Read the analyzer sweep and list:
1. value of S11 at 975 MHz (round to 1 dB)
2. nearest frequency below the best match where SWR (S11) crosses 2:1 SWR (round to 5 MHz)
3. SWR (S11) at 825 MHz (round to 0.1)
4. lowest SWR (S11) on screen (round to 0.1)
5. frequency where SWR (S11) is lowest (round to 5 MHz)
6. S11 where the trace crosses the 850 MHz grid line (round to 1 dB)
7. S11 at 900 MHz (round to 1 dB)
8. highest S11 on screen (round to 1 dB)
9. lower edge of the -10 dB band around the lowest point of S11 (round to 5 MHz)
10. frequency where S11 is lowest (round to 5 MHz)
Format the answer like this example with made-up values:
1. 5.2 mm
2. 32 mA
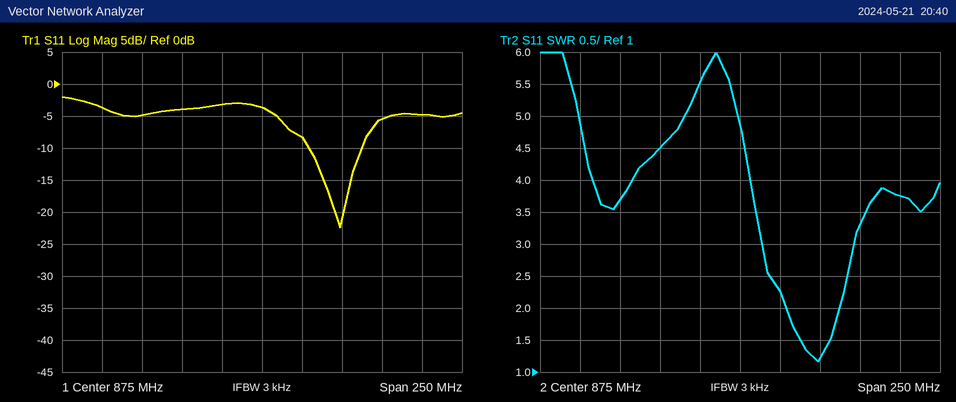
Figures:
1. -5 dB
2. 905 MHz
3. 4.5
4. 1.2
5. 925 MHz
6. -3 dB
7. -8 dB
8. -2 dB
9. 905 MHz
10. 925 MHz
